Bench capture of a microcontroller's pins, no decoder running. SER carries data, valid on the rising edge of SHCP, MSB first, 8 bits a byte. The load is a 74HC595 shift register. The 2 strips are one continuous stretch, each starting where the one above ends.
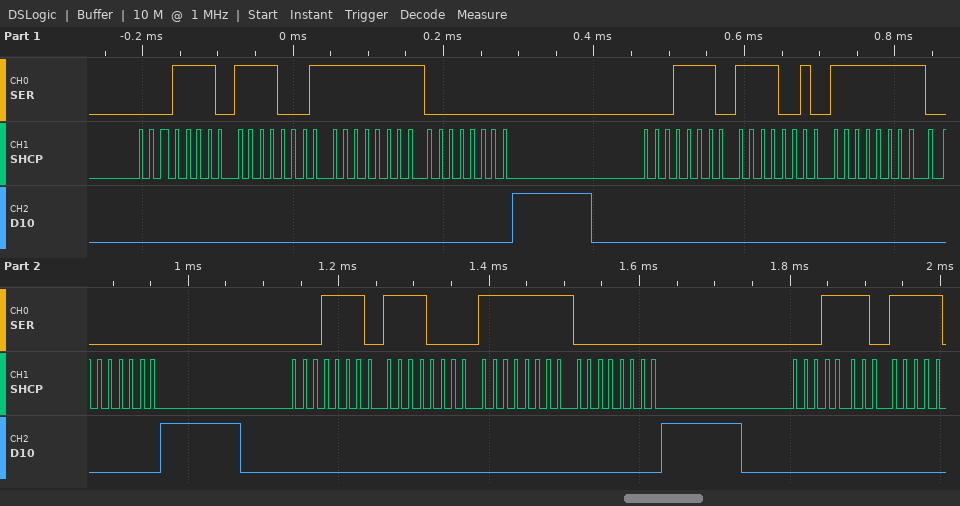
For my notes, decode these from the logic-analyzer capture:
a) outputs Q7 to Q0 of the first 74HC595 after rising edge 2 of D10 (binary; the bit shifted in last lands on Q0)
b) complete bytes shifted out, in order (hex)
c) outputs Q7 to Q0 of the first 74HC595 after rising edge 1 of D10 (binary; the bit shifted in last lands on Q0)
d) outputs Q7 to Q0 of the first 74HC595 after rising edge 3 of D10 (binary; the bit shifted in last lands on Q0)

00000000
0x1E 0xF1 0xFF 0x00 0x1E 0xF2 0xFF 0x00 0x1E 0xF0 0xFF 0x00 0x1E
00000000
00000000
